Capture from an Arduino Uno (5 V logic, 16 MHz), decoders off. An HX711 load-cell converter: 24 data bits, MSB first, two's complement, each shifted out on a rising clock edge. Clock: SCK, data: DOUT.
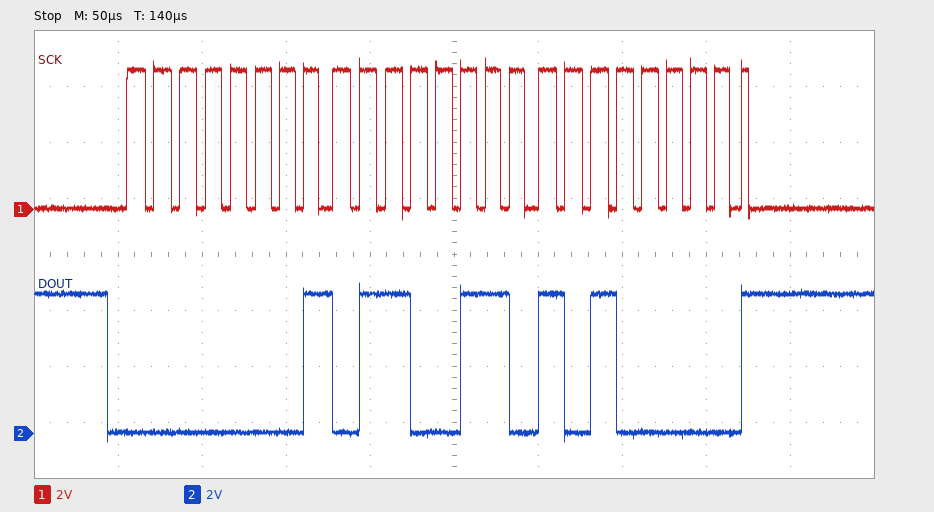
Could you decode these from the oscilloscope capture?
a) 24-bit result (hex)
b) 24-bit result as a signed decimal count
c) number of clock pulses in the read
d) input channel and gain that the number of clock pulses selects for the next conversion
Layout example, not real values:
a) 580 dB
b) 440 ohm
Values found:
a) 0x0166A0
b) 91808
c) 25
d) channel A, gain 128
